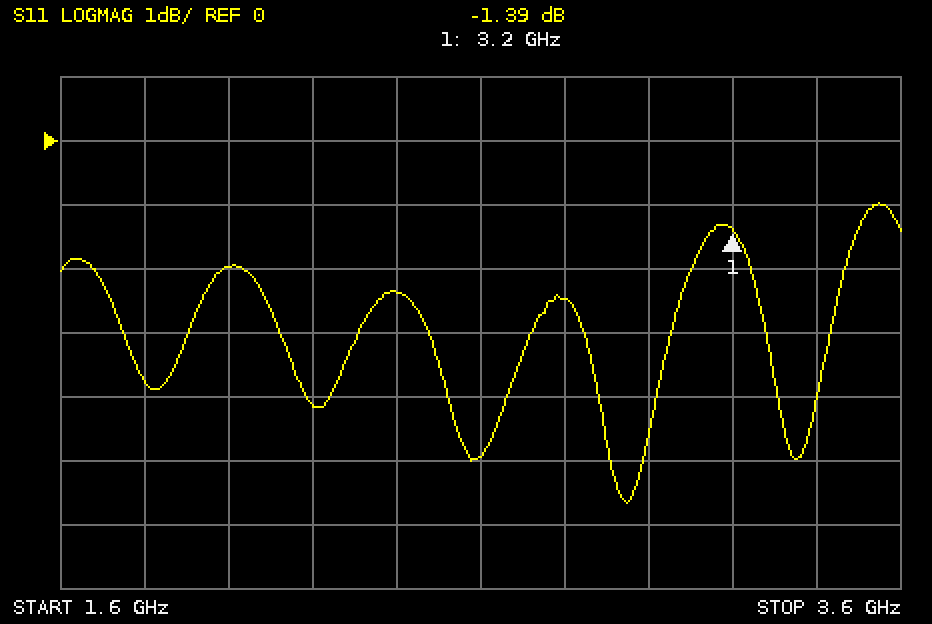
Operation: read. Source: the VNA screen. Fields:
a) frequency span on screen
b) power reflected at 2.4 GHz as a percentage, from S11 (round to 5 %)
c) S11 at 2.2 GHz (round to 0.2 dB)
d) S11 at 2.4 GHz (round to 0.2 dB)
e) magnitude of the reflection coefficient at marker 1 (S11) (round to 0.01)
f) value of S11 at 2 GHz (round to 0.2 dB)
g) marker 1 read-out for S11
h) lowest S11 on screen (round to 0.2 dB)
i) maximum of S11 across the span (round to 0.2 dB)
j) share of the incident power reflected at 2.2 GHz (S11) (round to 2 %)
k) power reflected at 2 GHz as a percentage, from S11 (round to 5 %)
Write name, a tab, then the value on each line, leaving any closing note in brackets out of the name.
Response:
frequency span on screen	2 GHz
power reflected at 2.4 GHz as a percentage, from S11	60 %
S11 at 2.2 GHz	-4.2 dB
S11 at 2.4 GHz	-2.4 dB
magnitude of the reflection coefficient at marker 1 (S11)	0.85
value of S11 at 2 GHz	-2.0 dB
marker 1 read-out for S11	-1.39 dB
lowest S11 on screen	-5.6 dB
maximum of S11 across the span	-1.0 dB
share of the incident power reflected at 2.2 GHz (S11)	38 %
power reflected at 2 GHz as a percentage, from S11	65 %
